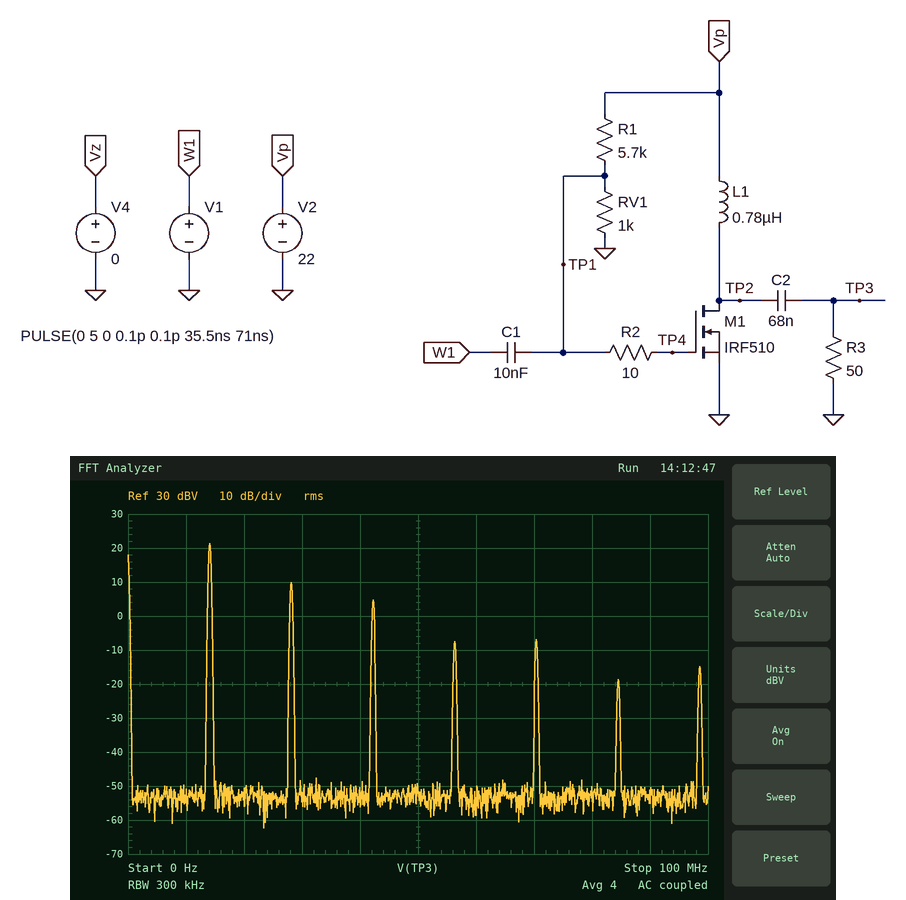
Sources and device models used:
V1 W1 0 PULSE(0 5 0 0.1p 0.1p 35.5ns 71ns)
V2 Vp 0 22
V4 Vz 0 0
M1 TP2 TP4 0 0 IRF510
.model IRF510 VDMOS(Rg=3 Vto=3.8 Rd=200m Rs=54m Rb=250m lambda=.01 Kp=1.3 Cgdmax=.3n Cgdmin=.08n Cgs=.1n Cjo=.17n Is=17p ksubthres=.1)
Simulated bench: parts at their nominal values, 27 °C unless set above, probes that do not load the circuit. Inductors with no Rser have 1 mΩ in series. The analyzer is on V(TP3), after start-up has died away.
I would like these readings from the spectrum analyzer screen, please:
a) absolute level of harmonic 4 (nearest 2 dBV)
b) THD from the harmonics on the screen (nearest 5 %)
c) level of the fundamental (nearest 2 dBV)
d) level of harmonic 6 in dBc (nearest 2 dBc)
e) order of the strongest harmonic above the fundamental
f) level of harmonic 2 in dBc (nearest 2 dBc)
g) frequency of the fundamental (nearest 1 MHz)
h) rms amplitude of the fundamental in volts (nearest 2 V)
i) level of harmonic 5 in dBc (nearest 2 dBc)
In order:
-8 dBV
30 %
22 dBV
-40 dBc
2
-12 dBc
14 MHz
12 V
-28 dBc
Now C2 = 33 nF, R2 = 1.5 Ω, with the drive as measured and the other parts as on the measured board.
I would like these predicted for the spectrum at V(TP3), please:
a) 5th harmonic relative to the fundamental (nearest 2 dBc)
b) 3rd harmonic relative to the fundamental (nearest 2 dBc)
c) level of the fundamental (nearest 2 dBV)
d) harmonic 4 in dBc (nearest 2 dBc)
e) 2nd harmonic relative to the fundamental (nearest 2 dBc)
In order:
-22 dBc
-14 dBc
26 dBV
-26 dBc
-14 dBc
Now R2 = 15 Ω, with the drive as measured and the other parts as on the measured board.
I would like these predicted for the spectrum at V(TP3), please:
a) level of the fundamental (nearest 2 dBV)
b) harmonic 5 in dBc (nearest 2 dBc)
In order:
20 dBV
-32 dBc
